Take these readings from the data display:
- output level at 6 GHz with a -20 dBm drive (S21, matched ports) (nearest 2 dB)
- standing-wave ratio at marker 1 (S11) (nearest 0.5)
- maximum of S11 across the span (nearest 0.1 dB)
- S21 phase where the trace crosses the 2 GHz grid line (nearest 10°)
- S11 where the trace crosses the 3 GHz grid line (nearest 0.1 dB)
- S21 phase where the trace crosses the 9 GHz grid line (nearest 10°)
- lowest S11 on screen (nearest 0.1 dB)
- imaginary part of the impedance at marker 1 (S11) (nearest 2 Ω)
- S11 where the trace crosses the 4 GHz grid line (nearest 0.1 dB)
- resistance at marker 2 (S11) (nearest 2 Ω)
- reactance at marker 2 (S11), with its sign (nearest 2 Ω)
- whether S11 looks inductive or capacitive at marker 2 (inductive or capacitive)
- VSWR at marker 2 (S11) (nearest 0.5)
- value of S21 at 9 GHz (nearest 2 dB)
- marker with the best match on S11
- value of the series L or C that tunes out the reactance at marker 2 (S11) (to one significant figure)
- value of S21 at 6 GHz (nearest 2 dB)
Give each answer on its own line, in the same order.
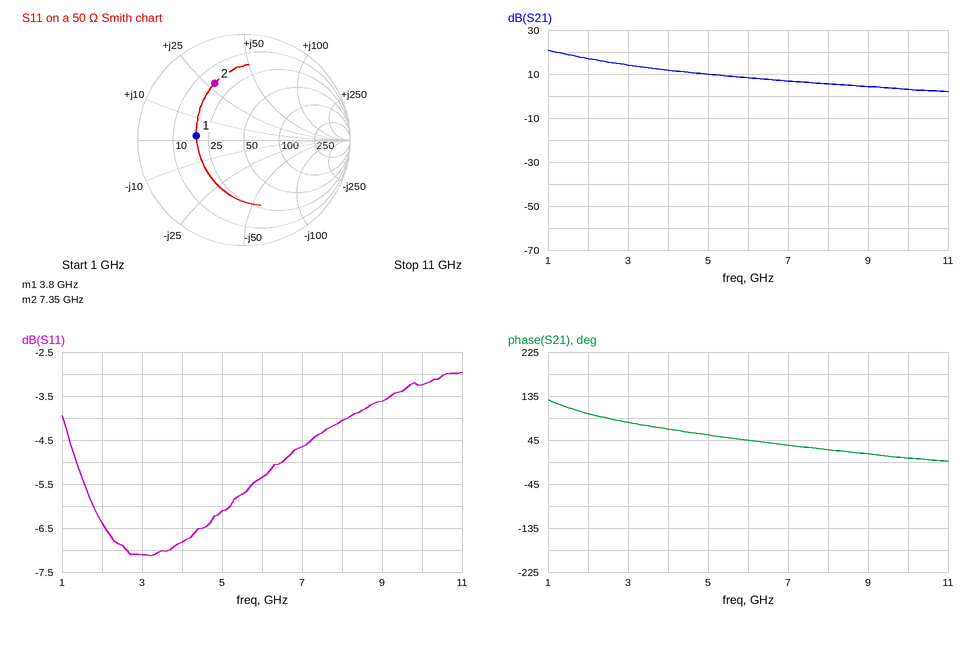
-12 dBm
2.5
-3.0 dB
100°
-7.1 dB
20°
-7.1 dB
+2 Ω
-6.8 dB
16 Ω
+28 Ω
inductive
4.0
4 dB
marker 1
800 fF
8 dB
